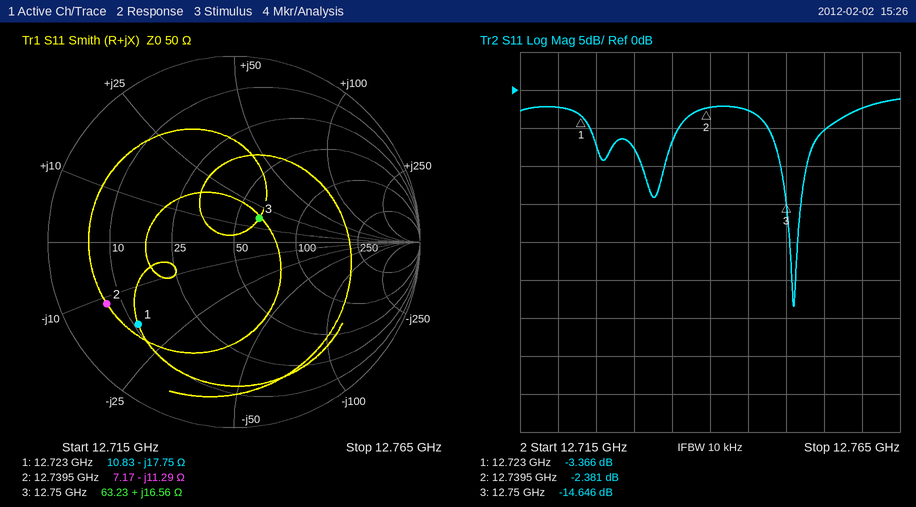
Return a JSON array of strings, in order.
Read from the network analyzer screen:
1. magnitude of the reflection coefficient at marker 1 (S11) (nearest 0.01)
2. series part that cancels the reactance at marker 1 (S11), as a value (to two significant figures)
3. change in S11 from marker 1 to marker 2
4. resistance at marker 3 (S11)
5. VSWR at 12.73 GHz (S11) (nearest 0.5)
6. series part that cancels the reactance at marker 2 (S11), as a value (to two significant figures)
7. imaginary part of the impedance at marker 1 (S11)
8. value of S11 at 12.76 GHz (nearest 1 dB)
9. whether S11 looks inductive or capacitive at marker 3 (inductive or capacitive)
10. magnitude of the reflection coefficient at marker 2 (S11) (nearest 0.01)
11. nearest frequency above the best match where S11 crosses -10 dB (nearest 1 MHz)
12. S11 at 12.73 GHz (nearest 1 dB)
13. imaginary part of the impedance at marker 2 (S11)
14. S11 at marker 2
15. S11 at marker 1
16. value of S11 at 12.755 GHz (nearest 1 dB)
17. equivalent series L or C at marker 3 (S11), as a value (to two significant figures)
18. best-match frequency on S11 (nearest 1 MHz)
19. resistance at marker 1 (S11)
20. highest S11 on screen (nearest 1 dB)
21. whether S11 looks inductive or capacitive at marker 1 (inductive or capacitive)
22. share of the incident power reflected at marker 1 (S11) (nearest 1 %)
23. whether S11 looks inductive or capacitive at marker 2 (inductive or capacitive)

["0.68", "220 pH", "0.985 dB", "63.23 Ω", "2.5", "140 pH", "-17.75 Ω", "-2 dB", "inductive", "0.76", "12.753 GHz", "-8 dB", "-11.29 Ω", "-2.381 dB", "-3.366 dB", "-5 dB", "210 pH", "12.751 GHz", "10.83 Ω", "-1 dB", "capacitive", "46 %", "capacitive"]
